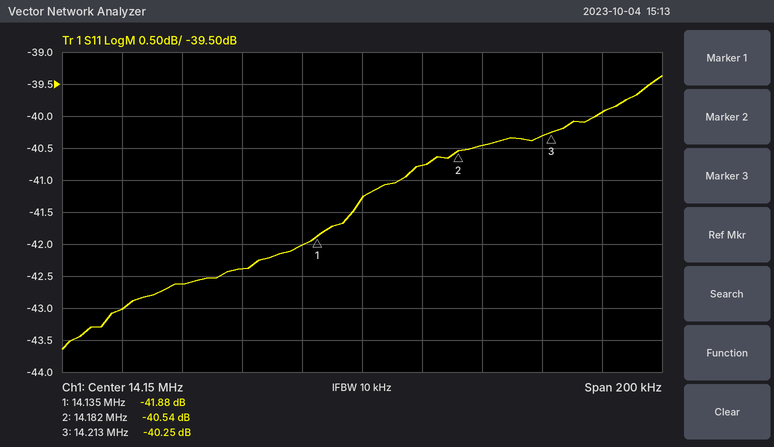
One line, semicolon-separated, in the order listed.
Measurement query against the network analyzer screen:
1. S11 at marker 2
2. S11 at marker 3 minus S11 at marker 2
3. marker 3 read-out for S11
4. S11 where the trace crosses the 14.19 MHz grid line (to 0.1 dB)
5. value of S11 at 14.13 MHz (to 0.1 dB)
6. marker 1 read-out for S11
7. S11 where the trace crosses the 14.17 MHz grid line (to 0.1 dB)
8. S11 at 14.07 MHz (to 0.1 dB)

-40.54 dB; 0.29 dB; -40.25 dB; -40.5 dB; -42.0 dB; -41.88 dB; -40.8 dB; -43.0 dB
